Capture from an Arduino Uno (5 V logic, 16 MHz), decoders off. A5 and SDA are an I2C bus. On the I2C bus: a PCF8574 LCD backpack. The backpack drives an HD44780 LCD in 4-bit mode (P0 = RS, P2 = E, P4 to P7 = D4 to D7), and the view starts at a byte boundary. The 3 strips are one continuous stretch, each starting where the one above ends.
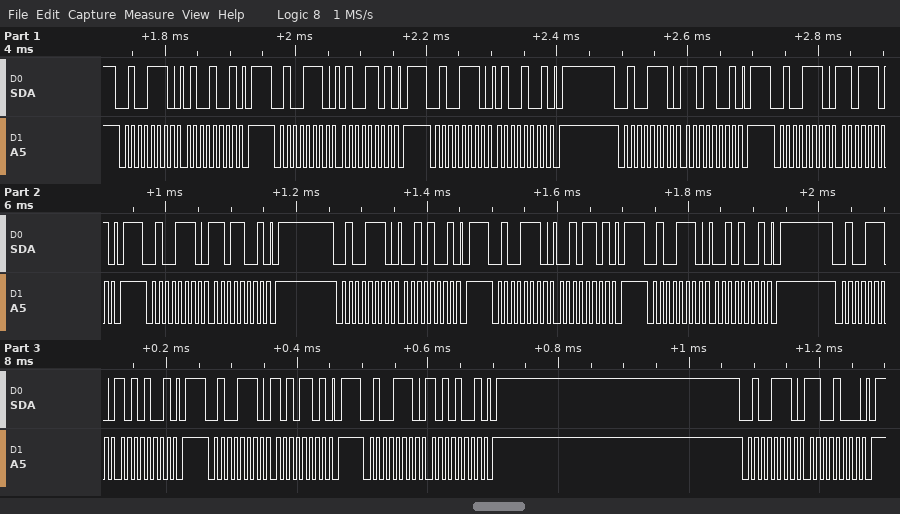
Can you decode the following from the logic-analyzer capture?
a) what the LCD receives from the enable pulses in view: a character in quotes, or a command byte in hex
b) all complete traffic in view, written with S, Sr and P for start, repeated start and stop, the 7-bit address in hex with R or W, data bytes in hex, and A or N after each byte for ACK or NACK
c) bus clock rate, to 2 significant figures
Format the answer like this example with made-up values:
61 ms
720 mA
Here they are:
'M' '*'
S 27W A 49 A P S 27W A 4D A P S 27W A 49 A P S 27W A D9 A P S 27W A DD A P S 27W A D9 A P S 27W A 29 A P S 27W A 2D A P S 27W A 29 A P S 27W A A9 A P S 27W A AD A P S 27W A A9 A P S 27W A C8 A P
100 kHz
